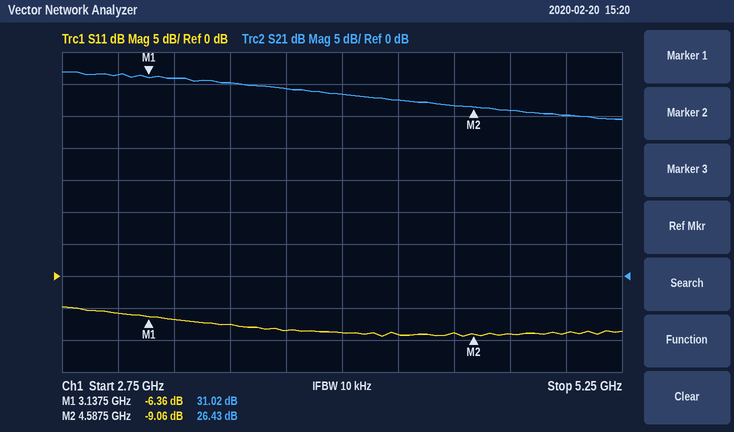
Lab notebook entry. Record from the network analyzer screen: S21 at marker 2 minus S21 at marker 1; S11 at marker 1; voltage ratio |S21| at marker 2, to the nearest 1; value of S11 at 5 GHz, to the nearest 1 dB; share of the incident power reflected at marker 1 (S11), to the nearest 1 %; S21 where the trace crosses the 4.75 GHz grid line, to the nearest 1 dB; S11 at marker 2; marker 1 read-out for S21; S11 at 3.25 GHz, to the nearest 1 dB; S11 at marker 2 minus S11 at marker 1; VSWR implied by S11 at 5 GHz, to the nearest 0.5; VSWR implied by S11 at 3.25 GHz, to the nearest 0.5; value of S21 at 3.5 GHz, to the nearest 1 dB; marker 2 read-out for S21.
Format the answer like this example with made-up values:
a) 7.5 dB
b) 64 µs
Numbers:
a) -4.59 dB
b) -6.36 dB
c) 21
d) -9 dB
e) 23 %
f) 26 dB
g) -9.06 dB
h) 31.02 dB
i) -7 dB
j) -2.70 dB
k) 2.0
l) 2.5
m) 30 dB
n) 26.43 dB
